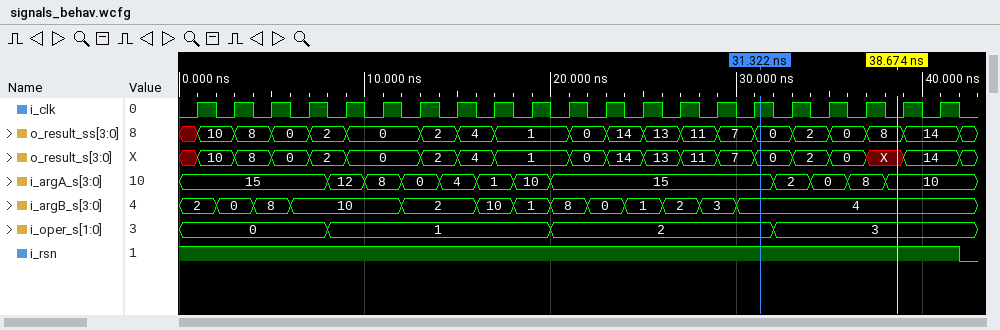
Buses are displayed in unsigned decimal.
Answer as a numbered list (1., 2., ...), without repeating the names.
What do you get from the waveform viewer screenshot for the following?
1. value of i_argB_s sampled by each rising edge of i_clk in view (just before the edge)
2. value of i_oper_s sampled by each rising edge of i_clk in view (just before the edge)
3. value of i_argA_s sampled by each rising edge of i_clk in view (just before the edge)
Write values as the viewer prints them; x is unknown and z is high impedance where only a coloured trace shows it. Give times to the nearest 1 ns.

1. 2, 0, 8, 10, 10, 10, 2, 2, 10, 1, 8, 0, 1, 2, 3, 4, 4, 4, 4, 4, 4
2. 0, 0, 0, 0, 1, 1, 1, 1, 1, 1, 2, 2, 2, 2, 2, 2, 3, 3, 3, 3, 3
3. 15, 15, 15, 15, 12, 8, 0, 4, 1, 10, 15, 15, 15, 15, 15, 15, 2, 0, 8, 10, 10
